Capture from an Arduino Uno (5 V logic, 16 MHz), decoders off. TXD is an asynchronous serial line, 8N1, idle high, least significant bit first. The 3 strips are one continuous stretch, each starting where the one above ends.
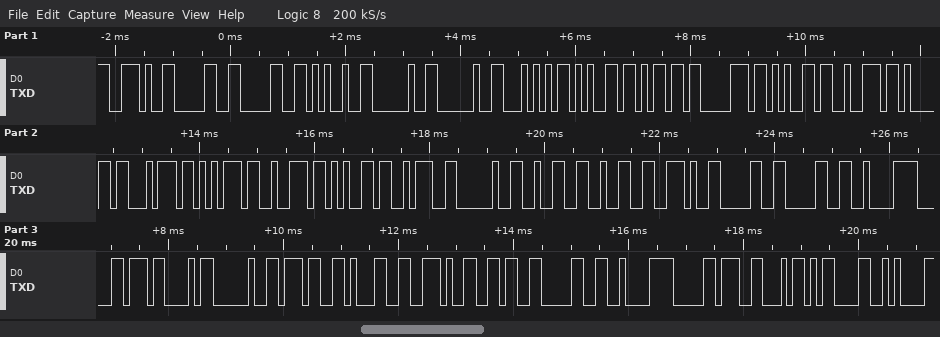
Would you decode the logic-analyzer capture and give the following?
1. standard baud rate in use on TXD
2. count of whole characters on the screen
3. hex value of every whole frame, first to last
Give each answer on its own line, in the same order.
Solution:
9600 baud
38
2E 30 30 25 20 20 54 65 6D 70 65 72 61 74 75 72 65 3A 20 32 32 2E 30 30 C2 B0 43 20 37 31 2E 36 30 C2 B0 46 0D 0A
